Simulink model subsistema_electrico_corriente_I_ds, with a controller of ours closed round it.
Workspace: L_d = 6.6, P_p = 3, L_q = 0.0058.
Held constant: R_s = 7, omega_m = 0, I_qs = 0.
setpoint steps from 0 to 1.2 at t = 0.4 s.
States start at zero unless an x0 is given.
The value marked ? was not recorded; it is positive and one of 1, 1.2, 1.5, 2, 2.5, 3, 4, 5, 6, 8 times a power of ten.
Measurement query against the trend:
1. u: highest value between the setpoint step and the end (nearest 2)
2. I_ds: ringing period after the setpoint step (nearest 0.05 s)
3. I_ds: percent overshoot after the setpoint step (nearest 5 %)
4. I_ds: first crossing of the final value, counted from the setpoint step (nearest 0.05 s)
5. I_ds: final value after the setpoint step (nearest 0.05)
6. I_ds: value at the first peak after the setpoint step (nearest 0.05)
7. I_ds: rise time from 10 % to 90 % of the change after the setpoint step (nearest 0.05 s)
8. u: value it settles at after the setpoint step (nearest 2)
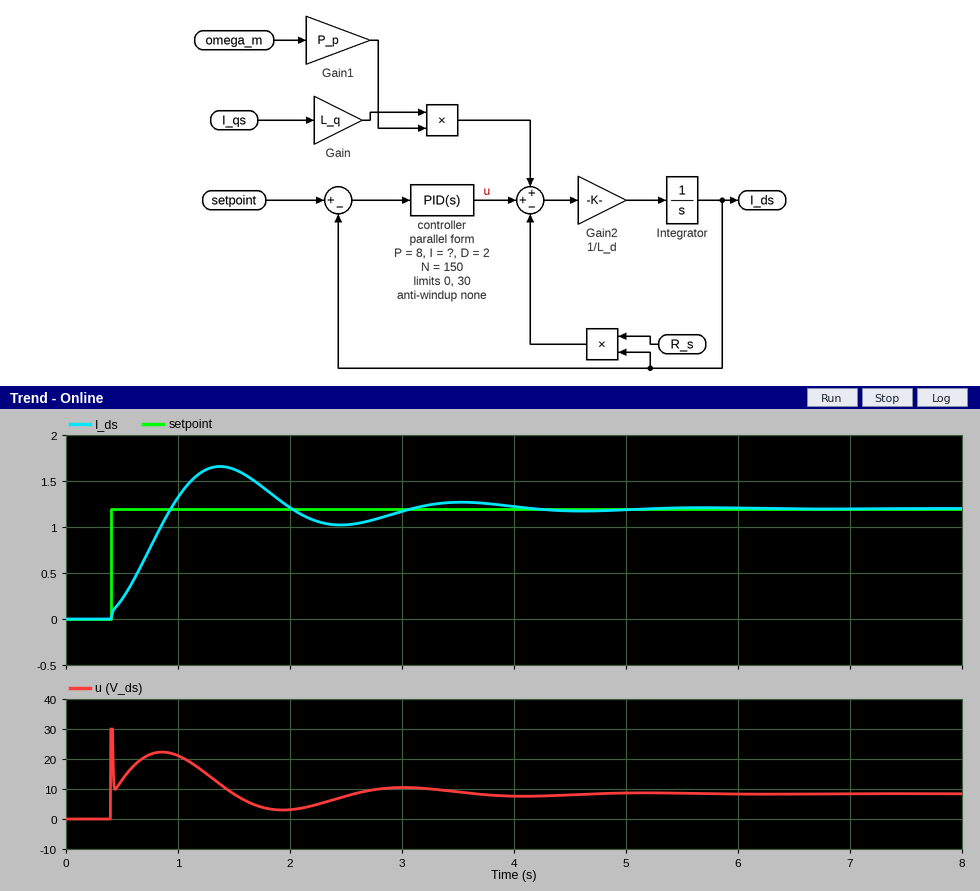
30
2.15 s
40 %
0.55 s
1.20
1.65
0.45 s
8
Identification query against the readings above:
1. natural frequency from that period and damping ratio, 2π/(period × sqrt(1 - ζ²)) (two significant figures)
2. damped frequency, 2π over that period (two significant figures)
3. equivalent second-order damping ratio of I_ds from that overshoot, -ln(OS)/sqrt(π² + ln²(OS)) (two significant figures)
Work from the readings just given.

3.0 rad/s
2.9 rad/s
0.28
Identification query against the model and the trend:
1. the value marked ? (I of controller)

80
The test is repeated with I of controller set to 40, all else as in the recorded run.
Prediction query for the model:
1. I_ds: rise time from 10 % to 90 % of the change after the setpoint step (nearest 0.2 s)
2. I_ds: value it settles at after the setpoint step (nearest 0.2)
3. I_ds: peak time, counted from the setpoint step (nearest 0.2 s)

0.6 s
1.2
1.4 s
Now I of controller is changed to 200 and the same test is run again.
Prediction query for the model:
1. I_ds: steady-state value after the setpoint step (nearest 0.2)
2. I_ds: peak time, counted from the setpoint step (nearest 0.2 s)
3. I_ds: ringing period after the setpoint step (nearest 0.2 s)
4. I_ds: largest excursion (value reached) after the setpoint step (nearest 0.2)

1.2
0.6 s
1.6 s
1.8
